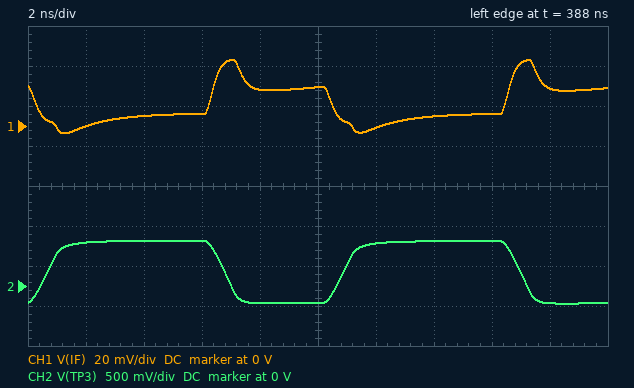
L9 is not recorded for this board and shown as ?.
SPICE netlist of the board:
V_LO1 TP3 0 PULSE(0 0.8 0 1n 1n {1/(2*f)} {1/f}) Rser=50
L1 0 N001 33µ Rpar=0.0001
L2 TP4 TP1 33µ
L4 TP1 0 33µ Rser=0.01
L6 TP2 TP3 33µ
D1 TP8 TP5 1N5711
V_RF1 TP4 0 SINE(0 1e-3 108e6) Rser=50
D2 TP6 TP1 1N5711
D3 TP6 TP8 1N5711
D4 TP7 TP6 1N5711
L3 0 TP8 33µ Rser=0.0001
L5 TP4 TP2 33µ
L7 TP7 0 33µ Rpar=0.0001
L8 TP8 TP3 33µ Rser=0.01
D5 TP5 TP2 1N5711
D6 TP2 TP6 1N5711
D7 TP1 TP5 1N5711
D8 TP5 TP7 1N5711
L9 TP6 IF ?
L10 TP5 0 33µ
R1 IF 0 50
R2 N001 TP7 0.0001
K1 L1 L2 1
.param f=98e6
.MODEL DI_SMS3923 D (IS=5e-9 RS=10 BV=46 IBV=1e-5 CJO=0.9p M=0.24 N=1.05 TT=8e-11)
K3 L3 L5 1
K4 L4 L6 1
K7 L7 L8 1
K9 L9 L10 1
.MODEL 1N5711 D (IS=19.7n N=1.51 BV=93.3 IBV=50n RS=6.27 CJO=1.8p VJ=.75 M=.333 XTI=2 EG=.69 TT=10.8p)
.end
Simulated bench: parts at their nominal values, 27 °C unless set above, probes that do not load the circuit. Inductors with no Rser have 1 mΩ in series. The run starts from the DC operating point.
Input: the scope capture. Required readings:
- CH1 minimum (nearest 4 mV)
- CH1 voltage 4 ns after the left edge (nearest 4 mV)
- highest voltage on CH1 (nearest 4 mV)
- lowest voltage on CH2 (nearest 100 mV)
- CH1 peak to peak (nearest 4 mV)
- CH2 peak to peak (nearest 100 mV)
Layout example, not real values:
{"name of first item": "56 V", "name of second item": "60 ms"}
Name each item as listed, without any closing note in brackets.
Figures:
{"CH1 minimum": "-4 mV", "CH1 voltage 4 ns after the left edge": "4 mV", "highest voltage on CH1": "32 mV", "lowest voltage on CH2": "-200 mV", "CH1 peak to peak": "36 mV", "CH2 peak to peak": "800 mV"}
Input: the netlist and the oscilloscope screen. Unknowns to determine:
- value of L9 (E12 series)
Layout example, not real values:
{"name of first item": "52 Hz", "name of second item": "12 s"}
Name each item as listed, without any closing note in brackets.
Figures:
{"value of L9": "56 µH"}
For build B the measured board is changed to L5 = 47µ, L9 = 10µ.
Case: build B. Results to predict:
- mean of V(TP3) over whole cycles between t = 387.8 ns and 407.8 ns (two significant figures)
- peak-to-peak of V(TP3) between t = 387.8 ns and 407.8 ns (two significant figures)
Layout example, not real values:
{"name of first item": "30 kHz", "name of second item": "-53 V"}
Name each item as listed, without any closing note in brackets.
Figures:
{"mean of V(TP3) over whole cycles between t = 387.8 ns and 407.8 ns": "7.5 mV", "peak-to-peak of V(TP3) between t = 387.8 ns and 407.8 ns": "13 mV"}
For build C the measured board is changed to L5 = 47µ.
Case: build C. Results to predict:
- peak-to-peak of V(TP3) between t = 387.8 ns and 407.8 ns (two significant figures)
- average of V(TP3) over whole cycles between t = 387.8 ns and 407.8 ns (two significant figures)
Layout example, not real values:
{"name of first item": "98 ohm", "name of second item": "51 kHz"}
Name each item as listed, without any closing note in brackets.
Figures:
{"peak-to-peak of V(TP3) between t = 387.8 ns and 407.8 ns": "13 mV", "average of V(TP3) over whole cycles between t = 387.8 ns and 407.8 ns": "7.5 mV"}
